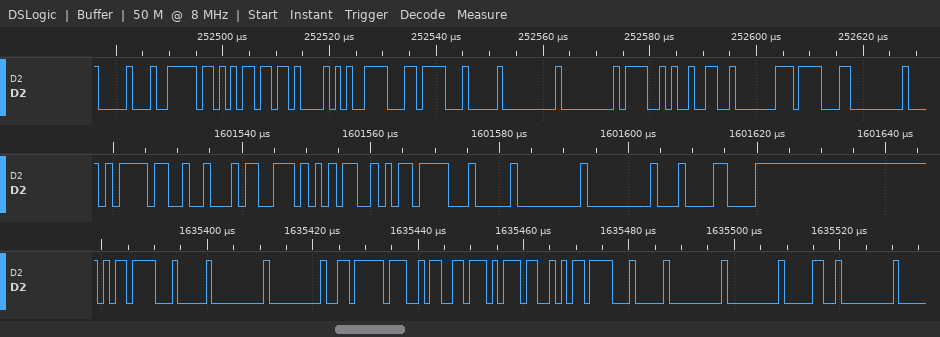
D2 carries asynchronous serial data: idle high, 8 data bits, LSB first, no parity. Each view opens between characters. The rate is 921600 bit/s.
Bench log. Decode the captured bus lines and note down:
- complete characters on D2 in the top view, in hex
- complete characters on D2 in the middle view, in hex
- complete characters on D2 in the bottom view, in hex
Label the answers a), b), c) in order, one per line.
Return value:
a) 10, BE, B5, 0B, E5, EC, 04, 00, 00, 4F, 32, C0, 8F, 00
b) BD, 12, 73, 35, ED, 04, 00, 00, 84, F8
c) ED, 04, 00, 00, F6, A7, 76, 37, ED, 04, 00, 00, 30, 00
